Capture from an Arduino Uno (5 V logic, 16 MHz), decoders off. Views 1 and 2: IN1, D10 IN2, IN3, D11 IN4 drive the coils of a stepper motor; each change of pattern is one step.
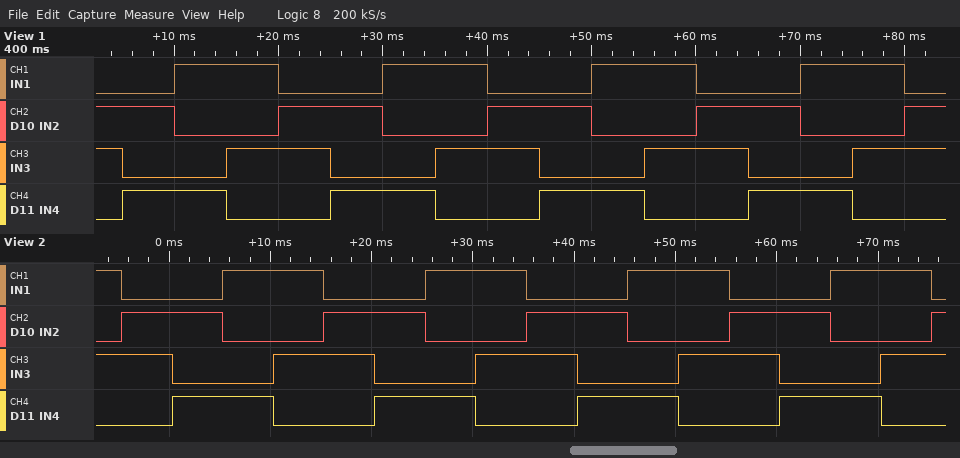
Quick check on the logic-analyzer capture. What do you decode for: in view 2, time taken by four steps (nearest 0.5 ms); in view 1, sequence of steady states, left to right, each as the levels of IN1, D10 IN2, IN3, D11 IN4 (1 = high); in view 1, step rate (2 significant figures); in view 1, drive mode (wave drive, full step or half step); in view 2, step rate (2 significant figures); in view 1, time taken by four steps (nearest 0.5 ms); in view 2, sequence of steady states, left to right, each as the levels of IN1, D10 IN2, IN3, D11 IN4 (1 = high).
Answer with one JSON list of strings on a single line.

["20.0 ms", "0110 0101 1001 1010 0110 0101 1001 1010 0110 0101 1001 1010 0110 0101 1001 1010 0110", "200 steps/s", "full step", "200 steps/s", "20.0 ms", "1010 0110 0101 1001 1010 0110 0101 1001 1010 0110 0101 1001 1010 0110 0101 1001 1010 0110"]
